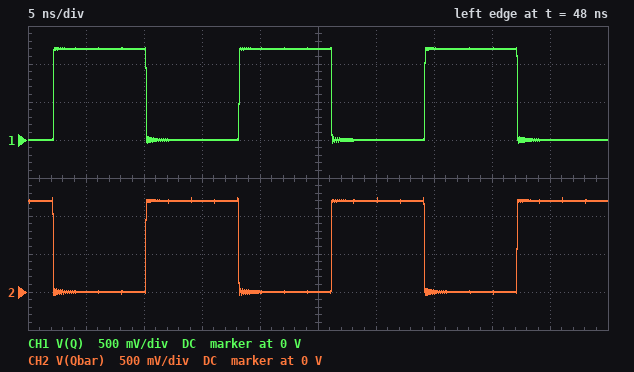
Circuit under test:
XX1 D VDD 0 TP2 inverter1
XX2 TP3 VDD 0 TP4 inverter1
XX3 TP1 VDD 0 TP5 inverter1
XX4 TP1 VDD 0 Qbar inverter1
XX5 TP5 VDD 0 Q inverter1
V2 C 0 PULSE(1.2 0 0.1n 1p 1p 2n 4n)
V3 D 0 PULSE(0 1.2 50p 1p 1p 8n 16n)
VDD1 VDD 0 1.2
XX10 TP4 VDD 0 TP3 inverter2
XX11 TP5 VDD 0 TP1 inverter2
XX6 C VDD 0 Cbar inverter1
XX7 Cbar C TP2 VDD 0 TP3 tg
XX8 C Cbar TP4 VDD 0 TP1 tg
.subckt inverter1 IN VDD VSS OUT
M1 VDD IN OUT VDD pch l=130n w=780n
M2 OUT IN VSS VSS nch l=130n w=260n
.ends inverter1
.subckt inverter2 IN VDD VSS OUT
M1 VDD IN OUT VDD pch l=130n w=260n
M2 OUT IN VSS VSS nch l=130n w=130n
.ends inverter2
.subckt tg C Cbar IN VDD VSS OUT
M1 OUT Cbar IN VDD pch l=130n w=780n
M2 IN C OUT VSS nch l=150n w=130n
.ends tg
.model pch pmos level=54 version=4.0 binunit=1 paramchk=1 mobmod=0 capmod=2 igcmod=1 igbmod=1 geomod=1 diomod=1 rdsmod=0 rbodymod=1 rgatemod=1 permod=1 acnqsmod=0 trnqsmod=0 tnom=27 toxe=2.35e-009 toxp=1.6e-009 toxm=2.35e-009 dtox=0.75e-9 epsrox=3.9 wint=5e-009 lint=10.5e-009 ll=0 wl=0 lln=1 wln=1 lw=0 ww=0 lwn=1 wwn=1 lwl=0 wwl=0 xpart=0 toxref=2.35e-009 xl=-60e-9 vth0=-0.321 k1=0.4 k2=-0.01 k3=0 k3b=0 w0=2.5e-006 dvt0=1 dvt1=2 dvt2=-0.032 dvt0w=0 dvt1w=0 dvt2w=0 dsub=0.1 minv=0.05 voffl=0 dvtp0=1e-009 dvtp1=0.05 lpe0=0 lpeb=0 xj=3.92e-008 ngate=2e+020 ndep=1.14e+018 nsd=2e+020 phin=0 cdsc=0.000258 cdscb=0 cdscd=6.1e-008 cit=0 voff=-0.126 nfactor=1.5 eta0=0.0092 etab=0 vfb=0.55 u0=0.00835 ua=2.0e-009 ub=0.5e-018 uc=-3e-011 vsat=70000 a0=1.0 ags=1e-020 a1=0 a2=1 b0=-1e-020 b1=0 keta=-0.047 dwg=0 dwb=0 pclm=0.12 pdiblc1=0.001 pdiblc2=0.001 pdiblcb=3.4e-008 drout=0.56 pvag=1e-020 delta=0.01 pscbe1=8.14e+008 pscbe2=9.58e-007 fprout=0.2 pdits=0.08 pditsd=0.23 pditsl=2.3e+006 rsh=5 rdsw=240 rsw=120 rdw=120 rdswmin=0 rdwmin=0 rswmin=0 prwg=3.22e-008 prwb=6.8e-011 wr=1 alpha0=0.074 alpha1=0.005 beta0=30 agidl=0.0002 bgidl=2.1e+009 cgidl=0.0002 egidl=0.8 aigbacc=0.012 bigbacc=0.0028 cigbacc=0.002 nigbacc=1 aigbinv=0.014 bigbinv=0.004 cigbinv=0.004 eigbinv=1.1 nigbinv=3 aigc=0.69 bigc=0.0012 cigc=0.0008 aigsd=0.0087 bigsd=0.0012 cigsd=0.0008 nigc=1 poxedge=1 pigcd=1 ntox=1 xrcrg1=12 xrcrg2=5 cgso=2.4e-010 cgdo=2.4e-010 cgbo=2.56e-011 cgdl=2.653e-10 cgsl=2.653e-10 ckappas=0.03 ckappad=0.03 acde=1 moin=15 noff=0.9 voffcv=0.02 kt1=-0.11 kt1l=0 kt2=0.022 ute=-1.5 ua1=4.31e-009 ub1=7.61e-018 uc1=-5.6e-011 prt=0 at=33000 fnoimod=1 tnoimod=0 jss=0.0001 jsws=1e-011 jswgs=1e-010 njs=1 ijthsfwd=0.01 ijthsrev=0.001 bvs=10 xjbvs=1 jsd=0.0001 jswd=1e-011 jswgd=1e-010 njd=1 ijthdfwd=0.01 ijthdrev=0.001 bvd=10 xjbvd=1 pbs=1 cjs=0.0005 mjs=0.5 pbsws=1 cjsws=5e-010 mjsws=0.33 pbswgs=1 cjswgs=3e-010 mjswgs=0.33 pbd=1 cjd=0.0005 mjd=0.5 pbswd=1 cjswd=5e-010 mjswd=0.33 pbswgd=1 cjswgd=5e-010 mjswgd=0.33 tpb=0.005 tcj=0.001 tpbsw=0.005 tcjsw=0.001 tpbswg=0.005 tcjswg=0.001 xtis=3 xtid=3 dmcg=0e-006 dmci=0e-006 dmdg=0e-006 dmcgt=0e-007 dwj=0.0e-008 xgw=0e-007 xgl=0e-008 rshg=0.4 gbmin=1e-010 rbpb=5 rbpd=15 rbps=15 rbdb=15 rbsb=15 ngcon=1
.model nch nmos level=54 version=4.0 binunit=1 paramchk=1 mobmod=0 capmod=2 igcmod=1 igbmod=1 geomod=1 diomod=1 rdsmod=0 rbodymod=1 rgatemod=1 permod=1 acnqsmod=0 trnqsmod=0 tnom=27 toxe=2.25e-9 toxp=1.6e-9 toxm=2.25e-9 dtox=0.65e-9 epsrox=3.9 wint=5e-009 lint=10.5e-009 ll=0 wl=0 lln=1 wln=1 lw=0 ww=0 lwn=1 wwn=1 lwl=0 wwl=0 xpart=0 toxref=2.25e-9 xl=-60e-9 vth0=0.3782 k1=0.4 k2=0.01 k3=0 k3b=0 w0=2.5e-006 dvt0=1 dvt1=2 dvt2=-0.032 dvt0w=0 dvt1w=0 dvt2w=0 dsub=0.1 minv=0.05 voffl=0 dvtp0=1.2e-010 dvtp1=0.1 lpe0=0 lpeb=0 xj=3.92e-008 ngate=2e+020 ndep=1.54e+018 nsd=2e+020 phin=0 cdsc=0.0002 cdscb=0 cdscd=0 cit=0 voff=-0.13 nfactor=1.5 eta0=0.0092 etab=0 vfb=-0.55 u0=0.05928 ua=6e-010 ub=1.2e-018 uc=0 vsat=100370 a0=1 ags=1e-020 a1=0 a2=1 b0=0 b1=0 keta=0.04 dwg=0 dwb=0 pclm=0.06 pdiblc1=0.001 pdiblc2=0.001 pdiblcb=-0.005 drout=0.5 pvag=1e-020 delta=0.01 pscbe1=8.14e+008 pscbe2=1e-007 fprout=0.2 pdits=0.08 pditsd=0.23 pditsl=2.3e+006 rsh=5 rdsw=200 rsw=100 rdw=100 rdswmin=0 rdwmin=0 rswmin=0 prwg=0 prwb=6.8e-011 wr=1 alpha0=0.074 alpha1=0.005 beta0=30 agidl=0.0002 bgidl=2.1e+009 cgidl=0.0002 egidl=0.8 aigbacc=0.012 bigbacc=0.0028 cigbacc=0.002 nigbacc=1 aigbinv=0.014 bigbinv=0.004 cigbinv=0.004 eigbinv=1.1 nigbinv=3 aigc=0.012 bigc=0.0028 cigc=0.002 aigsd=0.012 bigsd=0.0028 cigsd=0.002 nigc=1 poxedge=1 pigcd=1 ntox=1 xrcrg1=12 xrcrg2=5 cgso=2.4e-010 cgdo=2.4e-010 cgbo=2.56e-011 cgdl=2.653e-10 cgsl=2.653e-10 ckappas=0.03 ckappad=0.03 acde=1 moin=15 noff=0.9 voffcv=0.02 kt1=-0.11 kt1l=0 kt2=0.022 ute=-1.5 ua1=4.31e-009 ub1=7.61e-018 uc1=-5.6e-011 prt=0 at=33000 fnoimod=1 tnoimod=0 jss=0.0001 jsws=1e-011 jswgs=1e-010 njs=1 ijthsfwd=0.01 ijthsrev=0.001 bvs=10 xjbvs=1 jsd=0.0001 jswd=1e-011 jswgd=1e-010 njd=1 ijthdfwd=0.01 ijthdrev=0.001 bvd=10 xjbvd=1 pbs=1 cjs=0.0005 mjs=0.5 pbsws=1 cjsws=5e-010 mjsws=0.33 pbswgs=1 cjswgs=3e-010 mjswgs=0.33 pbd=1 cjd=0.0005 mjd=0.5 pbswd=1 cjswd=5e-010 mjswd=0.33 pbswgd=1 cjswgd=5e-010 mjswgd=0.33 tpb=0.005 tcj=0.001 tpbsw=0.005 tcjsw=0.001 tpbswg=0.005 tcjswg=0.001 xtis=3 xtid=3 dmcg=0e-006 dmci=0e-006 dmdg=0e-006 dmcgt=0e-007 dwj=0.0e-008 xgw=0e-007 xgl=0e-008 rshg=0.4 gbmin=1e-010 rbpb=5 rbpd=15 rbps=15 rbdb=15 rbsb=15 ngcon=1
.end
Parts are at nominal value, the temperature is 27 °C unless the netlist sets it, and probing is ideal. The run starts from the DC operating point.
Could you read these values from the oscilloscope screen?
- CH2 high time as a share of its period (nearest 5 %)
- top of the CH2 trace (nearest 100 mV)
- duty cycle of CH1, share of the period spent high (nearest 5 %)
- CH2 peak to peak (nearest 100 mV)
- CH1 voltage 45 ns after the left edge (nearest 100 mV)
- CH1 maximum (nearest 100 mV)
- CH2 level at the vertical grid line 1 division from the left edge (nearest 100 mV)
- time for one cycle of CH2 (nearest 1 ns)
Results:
50 %
1.2 V
50 %
1.3 V
0 V
1.2 V
0 V
16 ns
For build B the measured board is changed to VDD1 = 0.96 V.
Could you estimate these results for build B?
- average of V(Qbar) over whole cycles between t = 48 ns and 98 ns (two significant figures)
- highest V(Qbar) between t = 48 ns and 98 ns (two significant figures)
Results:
480 mV
990 mV
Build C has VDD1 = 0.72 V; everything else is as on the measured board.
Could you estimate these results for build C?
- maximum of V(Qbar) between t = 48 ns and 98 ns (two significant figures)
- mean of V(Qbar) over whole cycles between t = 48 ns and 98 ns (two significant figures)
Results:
750 mV
360 mV
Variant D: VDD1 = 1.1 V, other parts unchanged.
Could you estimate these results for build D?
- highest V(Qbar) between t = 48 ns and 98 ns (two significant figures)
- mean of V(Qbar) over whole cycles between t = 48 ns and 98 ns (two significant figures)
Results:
1.1 V
550 mV
